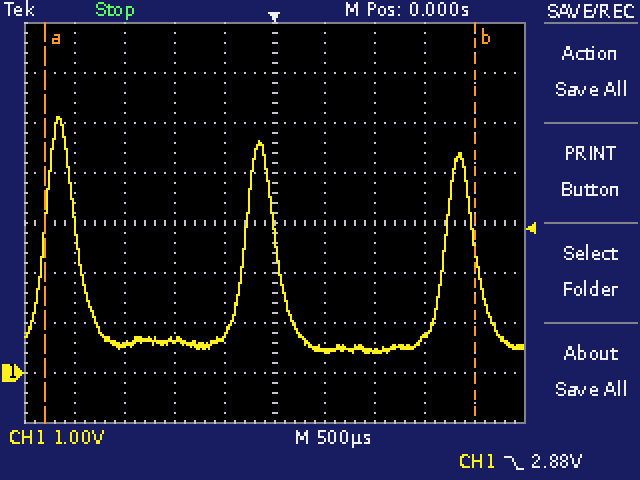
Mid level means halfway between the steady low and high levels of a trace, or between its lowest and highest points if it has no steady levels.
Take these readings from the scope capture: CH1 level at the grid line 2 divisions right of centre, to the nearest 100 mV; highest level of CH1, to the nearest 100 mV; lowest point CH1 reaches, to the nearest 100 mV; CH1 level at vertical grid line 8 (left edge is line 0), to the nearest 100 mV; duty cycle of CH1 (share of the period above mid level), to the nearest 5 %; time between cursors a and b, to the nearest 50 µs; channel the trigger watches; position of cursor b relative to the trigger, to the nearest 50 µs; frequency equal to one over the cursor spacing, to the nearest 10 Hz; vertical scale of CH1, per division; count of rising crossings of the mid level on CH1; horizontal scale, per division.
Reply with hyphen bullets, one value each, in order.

- 400 mV
- 5.1 V
- 400 mV
- 700 mV
- 15 %
- 4.30 ms
- CH1
- +2.00 ms
- 230 Hz
- 1 V
- 3
- 500 µs
